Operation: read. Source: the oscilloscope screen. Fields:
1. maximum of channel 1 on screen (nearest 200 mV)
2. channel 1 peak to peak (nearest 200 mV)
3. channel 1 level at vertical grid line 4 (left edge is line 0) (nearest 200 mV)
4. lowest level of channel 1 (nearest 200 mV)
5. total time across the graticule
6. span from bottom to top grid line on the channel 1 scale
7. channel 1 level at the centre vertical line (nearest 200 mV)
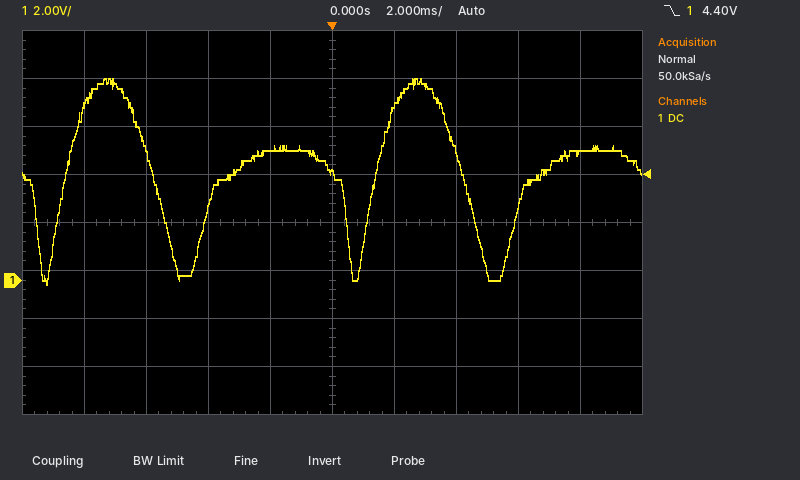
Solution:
8.4 V
8.6 V
5.4 V
-200 mV
20 ms
16 V
4.4 V
